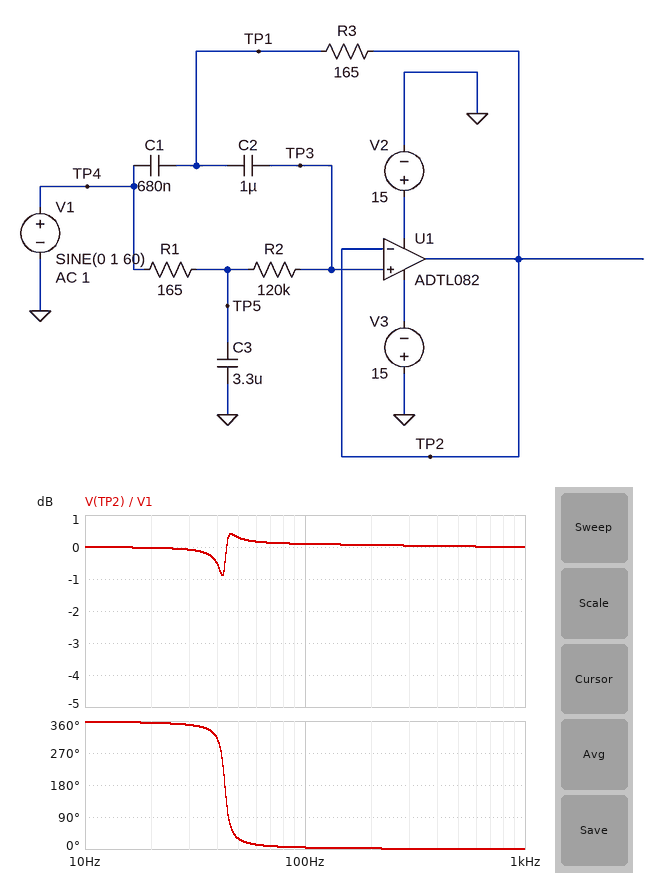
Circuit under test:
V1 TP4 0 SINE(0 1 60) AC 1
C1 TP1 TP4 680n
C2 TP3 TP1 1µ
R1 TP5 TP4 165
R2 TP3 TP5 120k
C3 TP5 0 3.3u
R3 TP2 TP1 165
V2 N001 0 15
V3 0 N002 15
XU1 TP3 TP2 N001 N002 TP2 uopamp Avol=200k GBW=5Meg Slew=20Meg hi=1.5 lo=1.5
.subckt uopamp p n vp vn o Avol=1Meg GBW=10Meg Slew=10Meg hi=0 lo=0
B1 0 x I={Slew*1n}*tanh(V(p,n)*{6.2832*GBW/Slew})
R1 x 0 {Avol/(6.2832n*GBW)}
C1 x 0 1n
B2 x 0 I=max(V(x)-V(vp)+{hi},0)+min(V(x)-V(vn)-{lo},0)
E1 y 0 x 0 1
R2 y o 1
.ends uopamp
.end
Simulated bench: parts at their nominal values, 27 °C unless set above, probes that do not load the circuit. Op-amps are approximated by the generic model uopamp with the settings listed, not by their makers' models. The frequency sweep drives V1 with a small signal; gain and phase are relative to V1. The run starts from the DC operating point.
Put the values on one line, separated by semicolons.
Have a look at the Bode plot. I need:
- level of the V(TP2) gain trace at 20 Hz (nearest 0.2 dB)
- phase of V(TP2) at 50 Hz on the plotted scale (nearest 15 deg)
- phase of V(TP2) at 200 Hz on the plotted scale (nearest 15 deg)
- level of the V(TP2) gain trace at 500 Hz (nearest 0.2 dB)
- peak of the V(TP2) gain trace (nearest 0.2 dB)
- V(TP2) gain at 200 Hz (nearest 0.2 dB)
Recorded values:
0 dB; 30 deg; 0 deg; 0 dB; 0.4 dB; 0 dB
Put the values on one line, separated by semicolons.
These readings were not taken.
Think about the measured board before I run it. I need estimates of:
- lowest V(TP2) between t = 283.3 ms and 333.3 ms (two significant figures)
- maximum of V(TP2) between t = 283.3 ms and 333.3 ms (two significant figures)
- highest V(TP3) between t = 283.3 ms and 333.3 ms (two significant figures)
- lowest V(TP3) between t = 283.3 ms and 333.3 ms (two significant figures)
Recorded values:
-1.0 V; 1.0 V; 1.0 V; -1.0 V
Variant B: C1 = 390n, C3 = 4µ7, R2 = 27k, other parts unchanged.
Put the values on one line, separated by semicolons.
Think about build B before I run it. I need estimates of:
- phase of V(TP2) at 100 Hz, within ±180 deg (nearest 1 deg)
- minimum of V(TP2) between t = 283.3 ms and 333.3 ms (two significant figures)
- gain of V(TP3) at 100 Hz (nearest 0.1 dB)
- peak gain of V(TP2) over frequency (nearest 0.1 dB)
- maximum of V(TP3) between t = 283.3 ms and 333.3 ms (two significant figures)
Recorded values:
-83 deg; -950 mV; -0.4 dB; 6.3 dB; 950 mV
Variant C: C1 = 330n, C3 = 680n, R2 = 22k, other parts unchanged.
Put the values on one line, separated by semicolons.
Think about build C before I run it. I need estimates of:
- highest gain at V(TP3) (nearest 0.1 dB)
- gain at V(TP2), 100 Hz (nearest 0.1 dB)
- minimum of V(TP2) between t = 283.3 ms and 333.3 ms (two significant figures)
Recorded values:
0 dB; -0.1 dB; -1.0 V
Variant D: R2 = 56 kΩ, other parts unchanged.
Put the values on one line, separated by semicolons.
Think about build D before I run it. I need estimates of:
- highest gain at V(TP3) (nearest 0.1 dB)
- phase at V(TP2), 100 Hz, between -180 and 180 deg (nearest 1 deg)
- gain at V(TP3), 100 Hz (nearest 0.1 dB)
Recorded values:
0.6 dB; 12 deg; 0.3 dB
